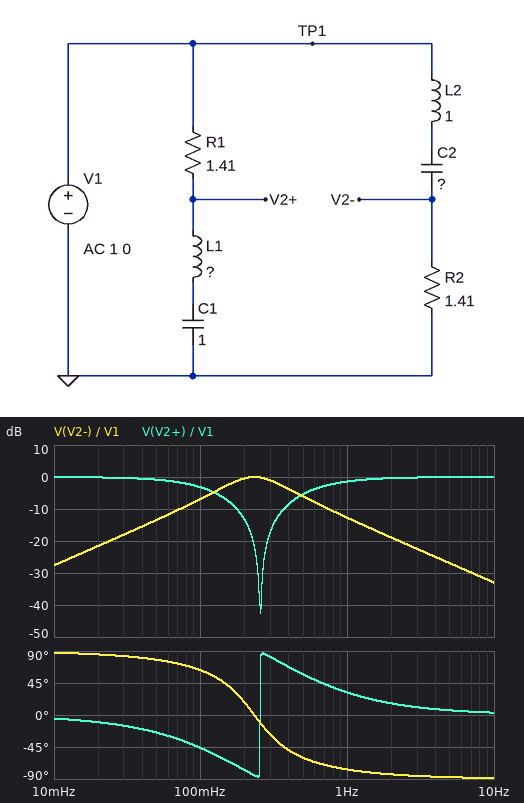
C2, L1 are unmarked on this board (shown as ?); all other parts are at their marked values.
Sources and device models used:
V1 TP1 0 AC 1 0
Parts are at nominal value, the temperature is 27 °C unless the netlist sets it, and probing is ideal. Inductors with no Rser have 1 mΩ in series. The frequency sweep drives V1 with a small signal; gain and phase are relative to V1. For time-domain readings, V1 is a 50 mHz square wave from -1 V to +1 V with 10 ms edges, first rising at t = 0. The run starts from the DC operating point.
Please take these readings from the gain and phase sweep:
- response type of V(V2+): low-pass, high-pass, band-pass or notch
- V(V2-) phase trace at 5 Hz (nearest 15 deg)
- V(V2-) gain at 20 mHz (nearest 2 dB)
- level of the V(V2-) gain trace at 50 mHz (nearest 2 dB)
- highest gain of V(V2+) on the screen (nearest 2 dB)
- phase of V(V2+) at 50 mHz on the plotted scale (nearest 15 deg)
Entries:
notch
-90 deg
-22 dB
-14 dB
0 dB
-30 deg
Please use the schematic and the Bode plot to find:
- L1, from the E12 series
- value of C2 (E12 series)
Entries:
390 mH
470 mF
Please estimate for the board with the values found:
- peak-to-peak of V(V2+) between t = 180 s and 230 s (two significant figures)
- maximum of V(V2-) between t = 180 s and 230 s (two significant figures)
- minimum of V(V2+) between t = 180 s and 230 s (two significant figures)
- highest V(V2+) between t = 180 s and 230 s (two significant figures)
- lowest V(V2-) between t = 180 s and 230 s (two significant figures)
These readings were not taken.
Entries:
2.0 V
1.1 V
-1.0 V
1.0 V
-1.1 V
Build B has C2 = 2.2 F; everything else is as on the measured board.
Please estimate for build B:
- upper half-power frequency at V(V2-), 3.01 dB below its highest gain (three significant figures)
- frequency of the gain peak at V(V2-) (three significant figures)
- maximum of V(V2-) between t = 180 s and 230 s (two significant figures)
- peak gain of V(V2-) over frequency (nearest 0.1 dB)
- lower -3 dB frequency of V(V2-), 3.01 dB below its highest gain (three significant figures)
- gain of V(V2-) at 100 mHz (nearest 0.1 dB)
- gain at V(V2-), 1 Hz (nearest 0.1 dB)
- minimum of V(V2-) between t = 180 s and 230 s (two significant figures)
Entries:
268 mHz
107 mHz
1.5 V
0 dB
43.0 mHz
0 dB
-13.1 dB
-1.5 V
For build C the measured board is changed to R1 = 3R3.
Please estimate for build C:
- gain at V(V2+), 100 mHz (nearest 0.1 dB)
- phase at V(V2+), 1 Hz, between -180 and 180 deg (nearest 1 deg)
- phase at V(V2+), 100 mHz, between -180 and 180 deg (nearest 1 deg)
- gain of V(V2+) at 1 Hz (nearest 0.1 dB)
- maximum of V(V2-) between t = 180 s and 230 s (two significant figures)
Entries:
-8.5 dB
55 deg
-68 deg
-4.9 dB
1.1 V
